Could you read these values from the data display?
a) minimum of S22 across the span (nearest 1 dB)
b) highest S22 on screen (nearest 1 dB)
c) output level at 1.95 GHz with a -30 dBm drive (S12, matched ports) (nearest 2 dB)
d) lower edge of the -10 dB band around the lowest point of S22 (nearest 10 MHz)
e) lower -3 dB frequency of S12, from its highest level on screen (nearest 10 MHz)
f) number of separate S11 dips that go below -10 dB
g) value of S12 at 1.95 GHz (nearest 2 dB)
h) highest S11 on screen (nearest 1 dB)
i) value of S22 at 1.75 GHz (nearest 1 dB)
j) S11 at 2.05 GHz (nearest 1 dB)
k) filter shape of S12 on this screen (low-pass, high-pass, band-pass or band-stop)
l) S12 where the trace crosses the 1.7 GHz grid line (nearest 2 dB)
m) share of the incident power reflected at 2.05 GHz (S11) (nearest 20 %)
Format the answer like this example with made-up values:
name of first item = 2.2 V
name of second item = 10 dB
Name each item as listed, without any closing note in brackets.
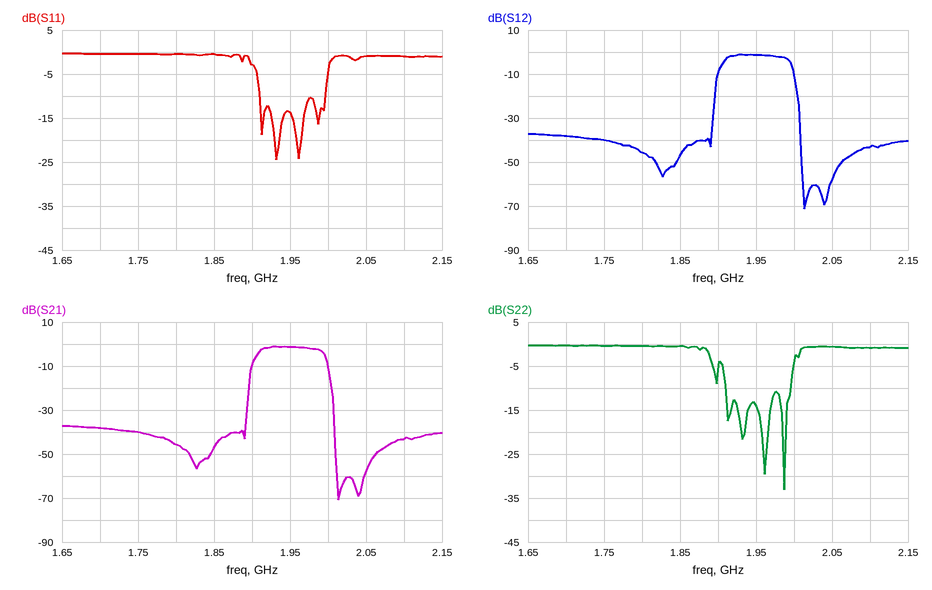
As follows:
minimum of S22 across the span = -33 dB
highest S22 on screen = 0 dB
output level at 1.95 GHz with a -30 dBm drive (S12, matched ports) = -32 dBm
lower edge of the -10 dB band around the lowest point of S22 = 1.91 GHz
lower -3 dB frequency of S12, from its highest level on screen = 1.91 GHz
number of separate S11 dips that go below -10 dB = 4
value of S12 at 1.95 GHz = -2 dB
highest S11 on screen = 0 dB
value of S22 at 1.75 GHz = 0 dB
S11 at 2.05 GHz = -1 dB
filter shape of S12 on this screen = band-pass
S12 where the trace crosses the 1.7 GHz grid line = -38 dB
share of the incident power reflected at 2.05 GHz (S11) = 80 %
